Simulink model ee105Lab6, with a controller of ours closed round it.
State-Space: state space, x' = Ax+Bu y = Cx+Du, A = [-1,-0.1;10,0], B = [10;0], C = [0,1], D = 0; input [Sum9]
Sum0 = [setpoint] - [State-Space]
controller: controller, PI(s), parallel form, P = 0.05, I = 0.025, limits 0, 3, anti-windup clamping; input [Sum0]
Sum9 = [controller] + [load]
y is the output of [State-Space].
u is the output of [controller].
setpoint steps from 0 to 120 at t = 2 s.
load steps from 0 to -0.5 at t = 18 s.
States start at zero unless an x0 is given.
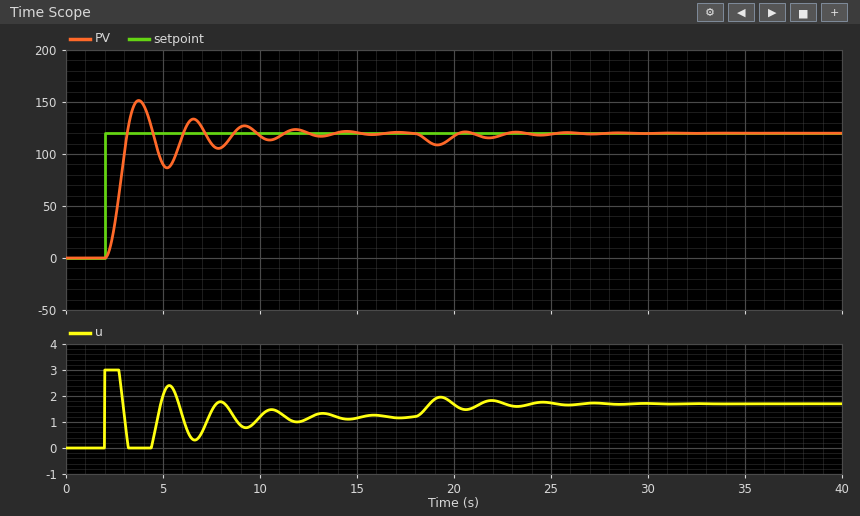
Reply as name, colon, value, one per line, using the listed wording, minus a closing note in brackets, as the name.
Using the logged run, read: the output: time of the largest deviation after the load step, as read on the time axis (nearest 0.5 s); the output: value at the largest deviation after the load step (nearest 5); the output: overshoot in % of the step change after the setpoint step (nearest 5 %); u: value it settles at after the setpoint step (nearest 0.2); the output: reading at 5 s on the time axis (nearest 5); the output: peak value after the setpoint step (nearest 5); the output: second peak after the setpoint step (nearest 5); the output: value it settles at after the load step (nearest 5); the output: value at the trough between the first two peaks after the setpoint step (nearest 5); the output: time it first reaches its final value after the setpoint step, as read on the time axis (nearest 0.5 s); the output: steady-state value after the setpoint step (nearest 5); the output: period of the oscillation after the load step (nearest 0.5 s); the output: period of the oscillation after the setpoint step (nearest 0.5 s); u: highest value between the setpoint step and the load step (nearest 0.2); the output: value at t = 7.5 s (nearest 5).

the output: time of the largest deviation after the load step, as read on the time axis: 19.0 s
the output: value at the largest deviation after the load step: 110
the output: overshoot in % of the step change after the setpoint step: 25 %
u: value it settles at after the setpoint step: 1.2
the output: reading at 5 s on the time axis: 90
the output: peak value after the setpoint step: 150
the output: second peak after the setpoint step: 135
the output: value it settles at after the load step: 120
the output: value at the trough between the first two peaks after the setpoint step: 85
the output: time it first reaches its final value after the setpoint step, as read on the time axis: 3.0 s
the output: steady-state value after the setpoint step: 120
the output: period of the oscillation after the load step: 2.5 s
the output: period of the oscillation after the setpoint step: 3.0 s
u: highest value between the setpoint step and the load step: 3.0
the output: value at t = 7.5 s: 110
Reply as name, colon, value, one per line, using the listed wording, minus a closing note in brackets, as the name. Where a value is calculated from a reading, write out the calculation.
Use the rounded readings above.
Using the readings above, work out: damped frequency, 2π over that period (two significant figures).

damped frequency, 2π over that period: 2π / 3 = 2.1 rad/s
